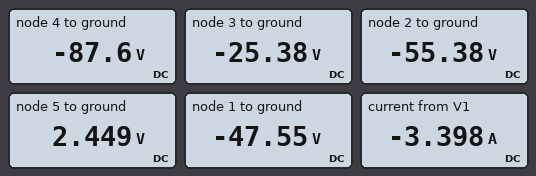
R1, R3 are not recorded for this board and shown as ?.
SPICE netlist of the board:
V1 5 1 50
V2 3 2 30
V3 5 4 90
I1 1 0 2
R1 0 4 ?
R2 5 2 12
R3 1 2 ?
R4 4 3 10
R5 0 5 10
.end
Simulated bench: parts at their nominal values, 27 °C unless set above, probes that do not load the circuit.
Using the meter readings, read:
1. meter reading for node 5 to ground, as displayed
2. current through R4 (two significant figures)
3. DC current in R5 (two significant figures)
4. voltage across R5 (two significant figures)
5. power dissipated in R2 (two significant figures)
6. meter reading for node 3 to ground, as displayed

2.449 V
6.2 A
240 mA
2.4 V
280 W
-25.38 V
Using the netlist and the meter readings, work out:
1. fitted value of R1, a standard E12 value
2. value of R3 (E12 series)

39 Ω
5.6 Ω
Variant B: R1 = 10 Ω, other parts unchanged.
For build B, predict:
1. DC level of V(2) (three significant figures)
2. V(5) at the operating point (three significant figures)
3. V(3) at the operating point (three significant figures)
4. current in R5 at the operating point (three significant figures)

-22.8 V
35.0 V
7.17 V
3.50 A
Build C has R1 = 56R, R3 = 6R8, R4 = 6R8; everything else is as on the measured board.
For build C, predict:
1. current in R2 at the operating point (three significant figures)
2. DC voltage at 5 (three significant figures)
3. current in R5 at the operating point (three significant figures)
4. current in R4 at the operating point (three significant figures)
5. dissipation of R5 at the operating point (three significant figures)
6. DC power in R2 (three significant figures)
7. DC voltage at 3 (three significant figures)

5.52 A
-3.33 V
333 mA
7.91 A
1.11 W
366 W
-39.6 V
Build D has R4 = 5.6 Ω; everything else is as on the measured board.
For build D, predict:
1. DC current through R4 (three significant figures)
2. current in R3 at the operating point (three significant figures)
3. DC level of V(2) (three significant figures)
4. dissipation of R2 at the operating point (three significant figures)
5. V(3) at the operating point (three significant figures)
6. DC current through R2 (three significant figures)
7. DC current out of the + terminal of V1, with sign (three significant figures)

9.12 A
3.38 A
-66.5 V
396 W
-36.5 V
5.74 A
-5.38 A
